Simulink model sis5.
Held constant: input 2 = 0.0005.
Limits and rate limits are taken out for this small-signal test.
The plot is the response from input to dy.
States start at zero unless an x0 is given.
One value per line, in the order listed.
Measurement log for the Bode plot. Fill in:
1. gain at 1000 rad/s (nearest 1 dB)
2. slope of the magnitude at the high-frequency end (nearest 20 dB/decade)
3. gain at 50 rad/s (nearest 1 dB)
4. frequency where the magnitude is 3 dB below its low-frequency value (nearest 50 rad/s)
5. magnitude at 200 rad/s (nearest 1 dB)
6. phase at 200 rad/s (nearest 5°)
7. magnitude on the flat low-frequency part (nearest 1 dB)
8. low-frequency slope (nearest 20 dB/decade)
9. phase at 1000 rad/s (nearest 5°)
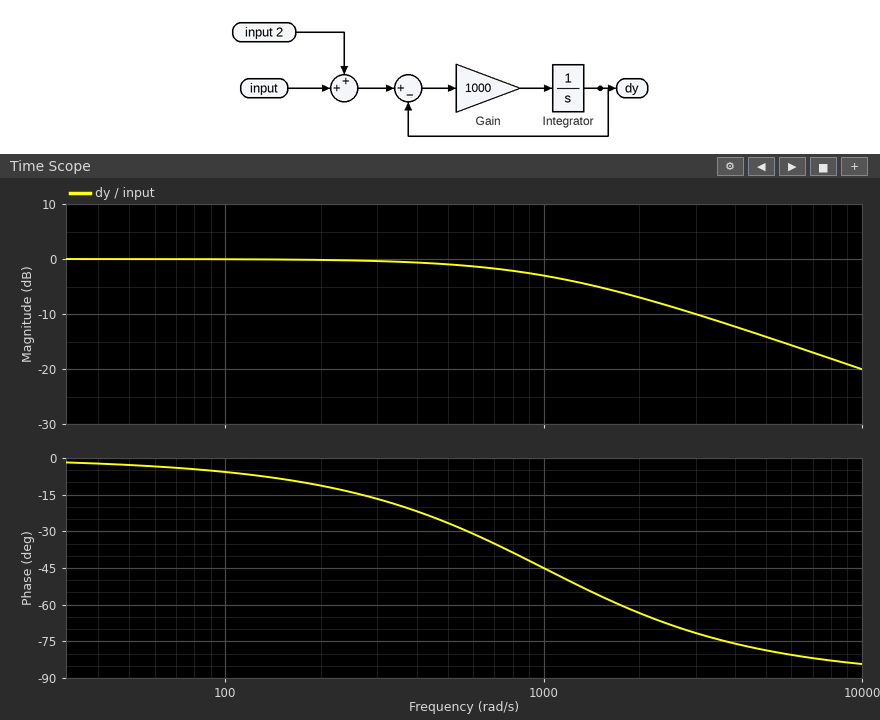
-3 dB
-20 dB/decade
0 dB
1000 rad/s
0 dB
-10°
0 dB
0 dB/decade
-45°
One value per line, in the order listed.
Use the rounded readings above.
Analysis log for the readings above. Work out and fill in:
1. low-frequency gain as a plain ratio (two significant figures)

1.0
